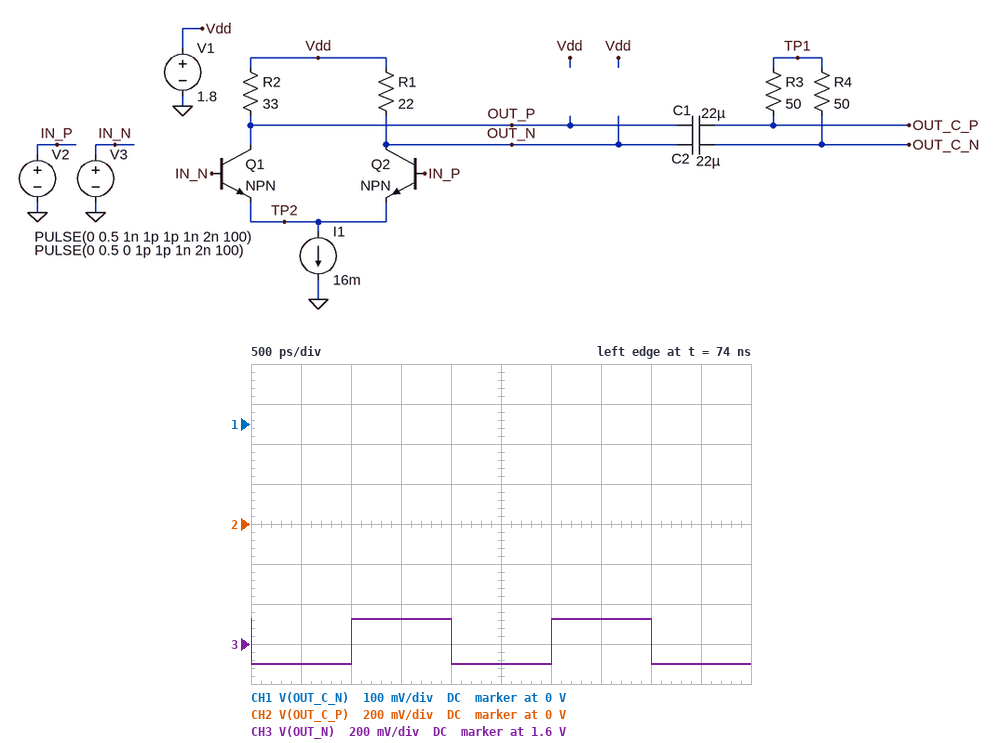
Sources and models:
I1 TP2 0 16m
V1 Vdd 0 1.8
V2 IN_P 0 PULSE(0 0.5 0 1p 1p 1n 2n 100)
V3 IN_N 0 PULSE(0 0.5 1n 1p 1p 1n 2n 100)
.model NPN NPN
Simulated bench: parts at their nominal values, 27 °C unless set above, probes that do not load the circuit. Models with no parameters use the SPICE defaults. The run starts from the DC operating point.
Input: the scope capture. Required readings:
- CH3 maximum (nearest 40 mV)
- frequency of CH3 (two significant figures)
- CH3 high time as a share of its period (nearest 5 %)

1.72 V
500 MHz
50 %
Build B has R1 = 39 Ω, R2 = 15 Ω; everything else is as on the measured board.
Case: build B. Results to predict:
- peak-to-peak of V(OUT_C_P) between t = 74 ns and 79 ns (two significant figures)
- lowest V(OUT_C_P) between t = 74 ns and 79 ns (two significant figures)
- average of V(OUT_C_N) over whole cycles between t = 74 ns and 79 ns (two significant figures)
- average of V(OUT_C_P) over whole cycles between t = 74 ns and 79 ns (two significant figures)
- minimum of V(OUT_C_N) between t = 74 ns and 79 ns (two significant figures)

150 mV
1.6 V
1.5 V
1.7 V
1.3 V
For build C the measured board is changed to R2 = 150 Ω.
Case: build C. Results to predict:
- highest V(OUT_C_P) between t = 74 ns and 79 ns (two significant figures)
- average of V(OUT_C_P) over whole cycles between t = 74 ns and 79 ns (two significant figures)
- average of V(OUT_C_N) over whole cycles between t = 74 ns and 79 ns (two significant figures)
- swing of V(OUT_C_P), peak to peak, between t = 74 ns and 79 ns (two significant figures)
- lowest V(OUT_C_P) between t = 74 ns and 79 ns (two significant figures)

1.6 V
1.2 V
1.5 V
870 mV
730 mV
